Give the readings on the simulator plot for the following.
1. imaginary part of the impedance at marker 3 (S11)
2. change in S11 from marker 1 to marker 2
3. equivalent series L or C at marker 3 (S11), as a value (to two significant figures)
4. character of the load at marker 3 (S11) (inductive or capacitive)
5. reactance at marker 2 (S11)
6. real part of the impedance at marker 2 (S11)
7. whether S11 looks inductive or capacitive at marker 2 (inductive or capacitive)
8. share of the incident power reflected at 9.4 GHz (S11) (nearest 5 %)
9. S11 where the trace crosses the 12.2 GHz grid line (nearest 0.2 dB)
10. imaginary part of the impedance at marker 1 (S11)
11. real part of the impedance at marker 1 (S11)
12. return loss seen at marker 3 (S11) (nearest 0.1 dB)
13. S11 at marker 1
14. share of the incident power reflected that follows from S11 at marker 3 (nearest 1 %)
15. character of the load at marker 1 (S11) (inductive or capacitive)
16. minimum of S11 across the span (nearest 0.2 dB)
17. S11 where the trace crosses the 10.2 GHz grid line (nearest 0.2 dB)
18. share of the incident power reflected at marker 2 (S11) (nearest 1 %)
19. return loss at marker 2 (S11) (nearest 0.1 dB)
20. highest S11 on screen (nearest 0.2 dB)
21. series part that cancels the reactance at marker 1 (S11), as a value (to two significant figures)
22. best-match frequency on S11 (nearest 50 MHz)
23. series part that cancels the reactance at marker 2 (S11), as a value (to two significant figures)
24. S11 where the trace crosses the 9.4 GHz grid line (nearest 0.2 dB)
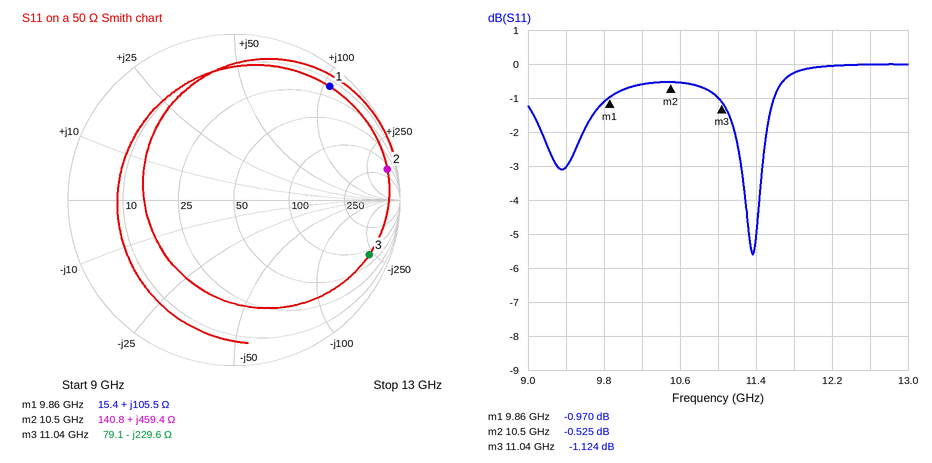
-229.6 Ω
0.445 dB
63 fF
capacitive
+459.4 Ω
140.8 Ω
inductive
50 %
0.0 dB
+105.5 Ω
15.4 Ω
1.1 dB
-0.970 dB
77 %
inductive
-5.6 dB
-0.6 dB
89 %
0.5 dB
0.0 dB
150 fF
11.35 GHz
33 fF
-3.0 dB
